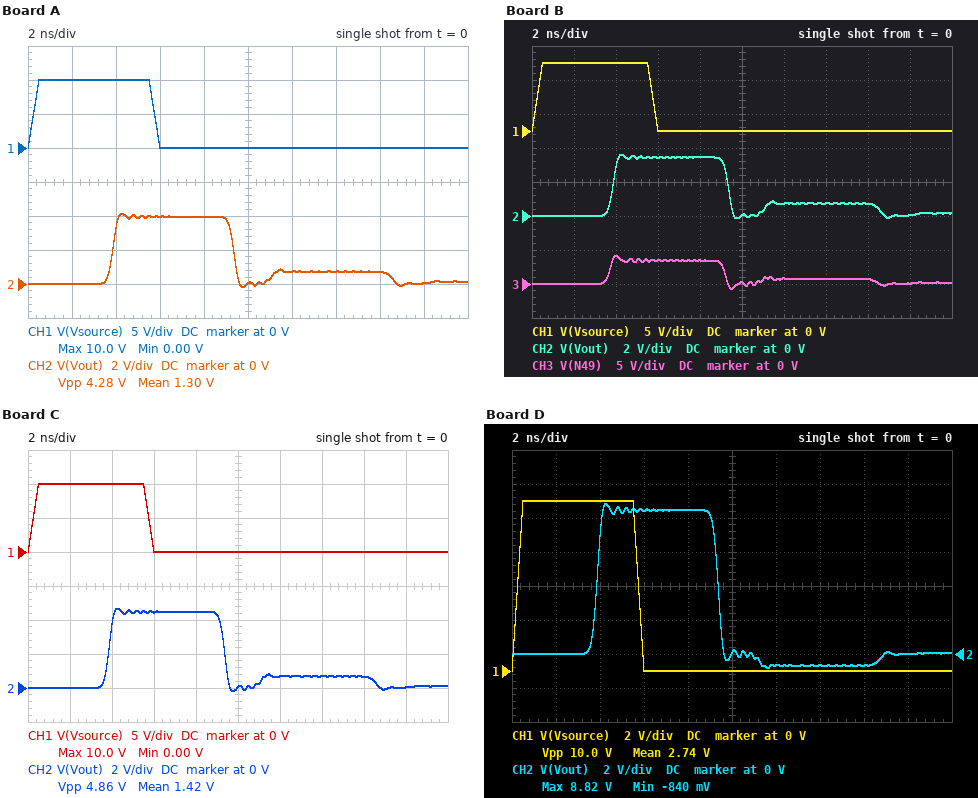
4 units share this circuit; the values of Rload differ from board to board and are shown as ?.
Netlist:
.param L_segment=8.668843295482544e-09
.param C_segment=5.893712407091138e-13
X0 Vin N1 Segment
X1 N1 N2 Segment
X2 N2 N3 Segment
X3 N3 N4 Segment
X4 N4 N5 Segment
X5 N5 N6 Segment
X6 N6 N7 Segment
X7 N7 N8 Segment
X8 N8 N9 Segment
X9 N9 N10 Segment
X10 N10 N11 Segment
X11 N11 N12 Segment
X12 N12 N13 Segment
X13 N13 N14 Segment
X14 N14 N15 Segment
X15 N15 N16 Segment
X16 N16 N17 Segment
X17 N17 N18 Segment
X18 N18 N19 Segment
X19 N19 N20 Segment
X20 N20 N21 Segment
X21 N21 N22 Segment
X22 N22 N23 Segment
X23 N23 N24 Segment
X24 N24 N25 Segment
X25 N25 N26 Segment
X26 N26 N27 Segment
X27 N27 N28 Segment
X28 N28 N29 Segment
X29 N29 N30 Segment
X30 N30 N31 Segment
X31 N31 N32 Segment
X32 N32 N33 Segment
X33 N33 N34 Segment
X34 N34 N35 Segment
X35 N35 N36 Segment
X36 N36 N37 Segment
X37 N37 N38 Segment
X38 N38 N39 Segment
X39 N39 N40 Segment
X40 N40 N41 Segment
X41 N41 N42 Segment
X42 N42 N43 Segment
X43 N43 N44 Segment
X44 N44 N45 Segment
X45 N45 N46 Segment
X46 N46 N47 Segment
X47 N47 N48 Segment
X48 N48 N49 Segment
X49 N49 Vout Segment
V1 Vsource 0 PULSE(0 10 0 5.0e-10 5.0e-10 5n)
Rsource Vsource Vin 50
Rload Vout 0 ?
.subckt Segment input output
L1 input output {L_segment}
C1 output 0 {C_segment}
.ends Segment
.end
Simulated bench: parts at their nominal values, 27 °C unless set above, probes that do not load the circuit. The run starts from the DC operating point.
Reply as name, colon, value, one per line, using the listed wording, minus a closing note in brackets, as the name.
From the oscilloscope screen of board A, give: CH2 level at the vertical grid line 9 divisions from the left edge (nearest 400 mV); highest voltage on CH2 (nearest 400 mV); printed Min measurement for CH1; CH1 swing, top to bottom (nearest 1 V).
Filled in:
CH2 level at the vertical grid line 9 divisions from the left edge: 0 V
highest voltage on CH2: 4.0 V
printed Min measurement for CH1: 0.00 V
CH1 swing, top to bottom: 10 V
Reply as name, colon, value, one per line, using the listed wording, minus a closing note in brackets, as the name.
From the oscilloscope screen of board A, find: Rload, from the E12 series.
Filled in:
Rload, from the E12 series: 47 Ω
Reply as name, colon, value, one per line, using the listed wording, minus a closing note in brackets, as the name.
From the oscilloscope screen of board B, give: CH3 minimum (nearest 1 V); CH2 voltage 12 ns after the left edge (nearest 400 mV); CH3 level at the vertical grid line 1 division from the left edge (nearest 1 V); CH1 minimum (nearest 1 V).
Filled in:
CH3 minimum: -1 V
CH2 voltage 12 ns after the left edge: 800 mV
CH3 level at the vertical grid line 1 division from the left edge: 0 V
CH1 minimum: 0 V
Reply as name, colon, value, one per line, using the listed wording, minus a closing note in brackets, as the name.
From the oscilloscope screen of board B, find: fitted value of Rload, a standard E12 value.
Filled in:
fitted value of Rload, a standard E12 value: 39 Ω
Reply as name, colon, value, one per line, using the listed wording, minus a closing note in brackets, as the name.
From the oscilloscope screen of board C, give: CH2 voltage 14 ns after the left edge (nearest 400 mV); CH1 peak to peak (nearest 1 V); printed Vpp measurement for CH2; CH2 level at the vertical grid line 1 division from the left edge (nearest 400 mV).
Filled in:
CH2 voltage 14 ns after the left edge: 800 mV
CH1 peak to peak: 10 V
printed Vpp measurement for CH2: 4.86 V
CH2 level at the vertical grid line 1 division from the left edge: 0 V
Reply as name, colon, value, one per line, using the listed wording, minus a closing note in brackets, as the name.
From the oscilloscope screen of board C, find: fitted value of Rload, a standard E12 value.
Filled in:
fitted value of Rload, a standard E12 value: 56 Ω
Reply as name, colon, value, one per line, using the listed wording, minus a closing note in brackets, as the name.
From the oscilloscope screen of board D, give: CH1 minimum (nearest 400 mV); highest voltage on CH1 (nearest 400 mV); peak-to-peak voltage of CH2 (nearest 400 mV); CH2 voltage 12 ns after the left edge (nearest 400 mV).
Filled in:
CH1 minimum: 0 V
highest voltage on CH1: 10.0 V
peak-to-peak voltage of CH2: 9.6 V
CH2 voltage 12 ns after the left edge: -800 mV
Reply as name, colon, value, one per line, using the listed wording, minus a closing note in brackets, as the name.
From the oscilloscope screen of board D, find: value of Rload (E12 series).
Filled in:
value of Rload: 180 Ω
